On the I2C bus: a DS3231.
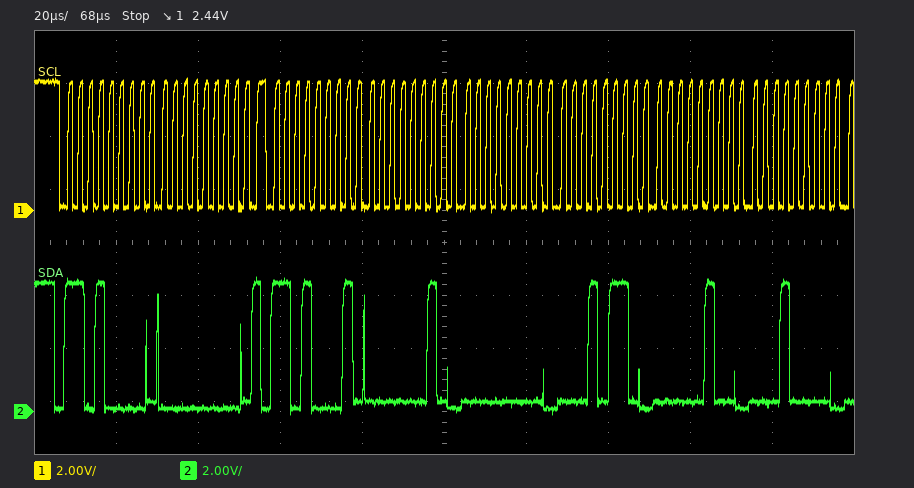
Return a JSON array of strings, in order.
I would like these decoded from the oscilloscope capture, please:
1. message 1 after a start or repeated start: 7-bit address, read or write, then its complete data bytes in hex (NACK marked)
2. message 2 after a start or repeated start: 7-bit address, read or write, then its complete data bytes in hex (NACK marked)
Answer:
["0x68 write: 00", "0x68 read: 02 00 16 04 10"]
